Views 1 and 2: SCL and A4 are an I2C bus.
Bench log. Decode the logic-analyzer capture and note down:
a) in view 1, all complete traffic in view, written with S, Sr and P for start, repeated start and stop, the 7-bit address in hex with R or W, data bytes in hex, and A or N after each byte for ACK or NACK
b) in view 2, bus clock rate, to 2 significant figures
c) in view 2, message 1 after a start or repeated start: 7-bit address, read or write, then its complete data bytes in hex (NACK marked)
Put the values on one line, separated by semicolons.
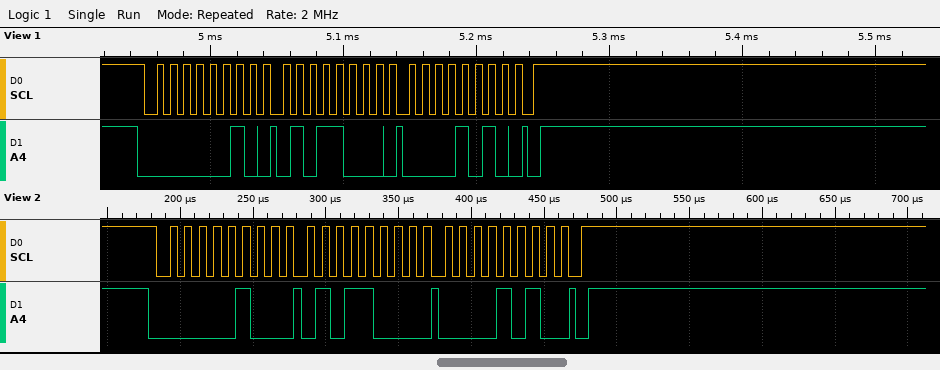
S 01W A 58 A 0A A P; 100 kHz; 0x02 write: 58 0A
